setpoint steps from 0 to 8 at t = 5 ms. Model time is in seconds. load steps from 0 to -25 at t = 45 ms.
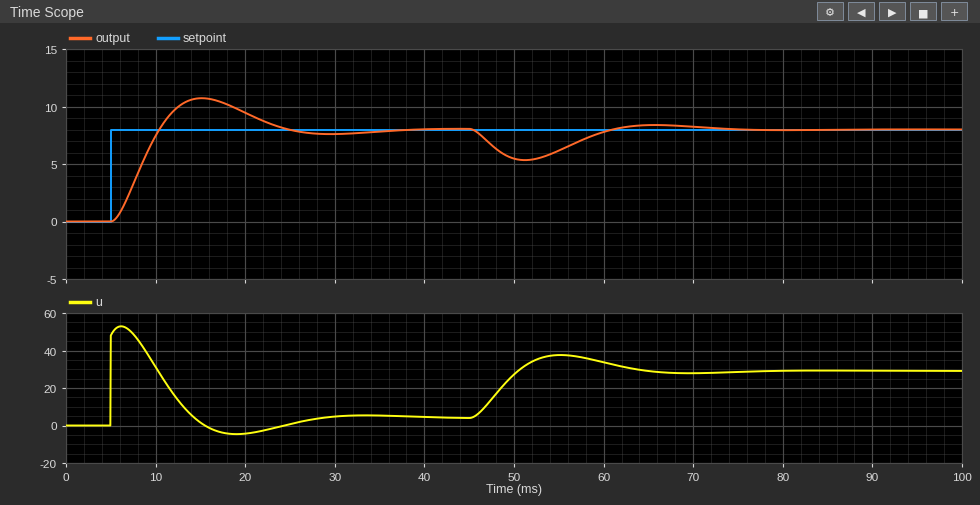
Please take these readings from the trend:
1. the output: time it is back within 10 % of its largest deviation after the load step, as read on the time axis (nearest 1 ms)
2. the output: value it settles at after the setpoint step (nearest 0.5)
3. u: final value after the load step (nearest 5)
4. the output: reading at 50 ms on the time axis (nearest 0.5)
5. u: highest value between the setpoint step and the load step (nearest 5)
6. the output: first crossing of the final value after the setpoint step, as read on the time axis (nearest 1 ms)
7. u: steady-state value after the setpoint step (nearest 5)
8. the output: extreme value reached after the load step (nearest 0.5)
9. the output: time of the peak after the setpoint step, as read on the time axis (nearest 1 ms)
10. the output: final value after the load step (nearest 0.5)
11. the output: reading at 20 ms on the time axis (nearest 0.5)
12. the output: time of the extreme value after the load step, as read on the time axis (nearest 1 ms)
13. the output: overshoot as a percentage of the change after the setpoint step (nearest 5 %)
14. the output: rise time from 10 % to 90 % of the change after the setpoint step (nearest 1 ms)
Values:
69 ms
8.0
30
5.5
55
10 ms
5
5.5
15 ms
8.0
9.5
51 ms
35 %
4 ms
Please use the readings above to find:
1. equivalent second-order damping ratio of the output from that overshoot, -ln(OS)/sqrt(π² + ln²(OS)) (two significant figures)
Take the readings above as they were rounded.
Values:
0.32
